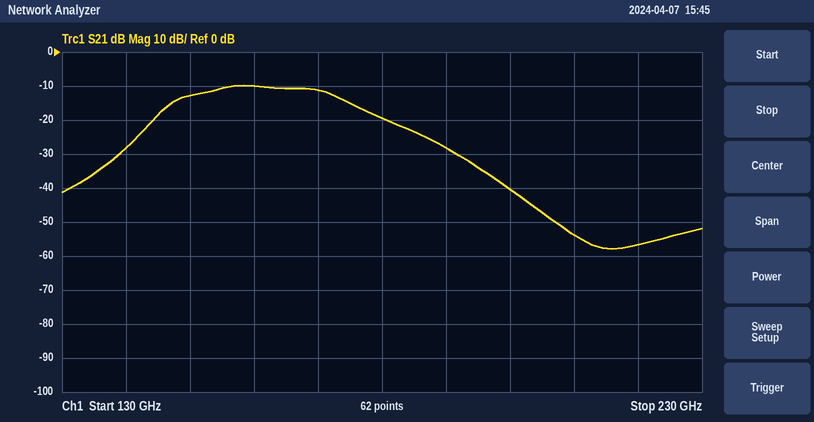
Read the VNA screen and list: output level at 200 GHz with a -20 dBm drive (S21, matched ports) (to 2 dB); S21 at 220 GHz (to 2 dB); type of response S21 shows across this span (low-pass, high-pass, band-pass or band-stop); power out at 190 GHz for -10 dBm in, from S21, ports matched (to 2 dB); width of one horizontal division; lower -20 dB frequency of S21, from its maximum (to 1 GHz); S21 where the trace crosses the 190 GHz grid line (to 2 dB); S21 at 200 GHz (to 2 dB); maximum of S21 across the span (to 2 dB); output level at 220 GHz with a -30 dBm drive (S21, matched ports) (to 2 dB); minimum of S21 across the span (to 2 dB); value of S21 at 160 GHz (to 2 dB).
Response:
-60 dBm
-56 dB
band-pass
-38 dBm
10 GHz
139 GHz
-28 dB
-40 dB
-10 dB
-86 dBm
-58 dB
-10 dB
